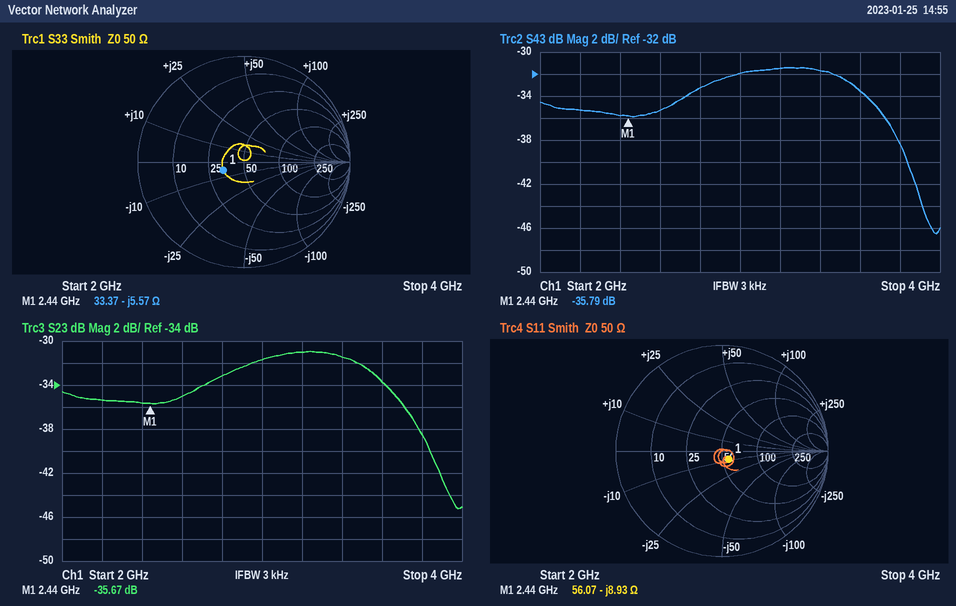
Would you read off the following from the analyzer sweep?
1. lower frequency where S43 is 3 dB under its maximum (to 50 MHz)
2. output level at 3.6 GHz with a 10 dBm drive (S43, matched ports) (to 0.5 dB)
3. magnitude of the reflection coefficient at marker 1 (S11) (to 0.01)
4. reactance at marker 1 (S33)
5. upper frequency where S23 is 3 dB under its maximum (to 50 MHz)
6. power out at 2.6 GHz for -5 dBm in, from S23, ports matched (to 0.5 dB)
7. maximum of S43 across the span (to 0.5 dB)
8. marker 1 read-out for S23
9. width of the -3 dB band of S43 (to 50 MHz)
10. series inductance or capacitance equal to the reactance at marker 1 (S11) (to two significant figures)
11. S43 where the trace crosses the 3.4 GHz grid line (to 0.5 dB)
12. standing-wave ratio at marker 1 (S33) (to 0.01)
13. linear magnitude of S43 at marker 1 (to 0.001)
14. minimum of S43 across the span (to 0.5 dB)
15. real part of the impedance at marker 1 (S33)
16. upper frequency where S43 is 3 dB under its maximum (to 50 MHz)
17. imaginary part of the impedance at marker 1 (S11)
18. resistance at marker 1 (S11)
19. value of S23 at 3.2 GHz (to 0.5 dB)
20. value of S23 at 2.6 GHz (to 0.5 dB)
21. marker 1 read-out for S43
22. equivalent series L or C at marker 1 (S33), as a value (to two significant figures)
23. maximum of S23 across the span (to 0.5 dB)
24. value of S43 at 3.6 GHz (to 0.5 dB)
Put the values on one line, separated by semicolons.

2.70 GHz; -23.5 dBm; 0.10; -5.57 Ω; 3.60 GHz; -40.0 dBm; -31.5 dB; -35.67 dB; 950 MHz; 7.3 pF; -31.5 dB; 1.53; 0.016; -46.5 dB; 33.37 Ω; 3.65 GHz; -8.93 Ω; 56.07 Ω; -31.0 dB; -35.0 dB; -35.79 dB; 12 pF; -31.0 dB; -33.5 dB
